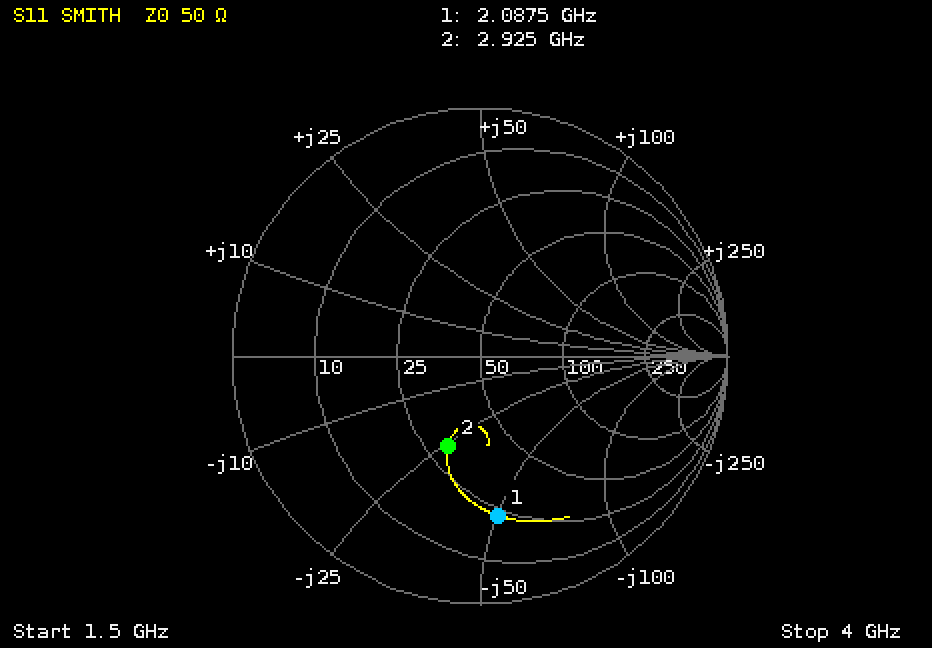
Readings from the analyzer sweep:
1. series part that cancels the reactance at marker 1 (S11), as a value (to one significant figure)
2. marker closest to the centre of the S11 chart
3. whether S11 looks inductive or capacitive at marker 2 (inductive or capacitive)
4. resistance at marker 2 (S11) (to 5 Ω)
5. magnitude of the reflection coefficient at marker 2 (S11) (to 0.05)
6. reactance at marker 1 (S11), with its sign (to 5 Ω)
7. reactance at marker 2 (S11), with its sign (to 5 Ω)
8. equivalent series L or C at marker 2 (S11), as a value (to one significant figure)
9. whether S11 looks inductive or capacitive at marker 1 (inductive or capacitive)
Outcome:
4 nH
marker 2
capacitive
30 Ω
0.40
-50 Ω
-25 Ω
2 pF
capacitive
